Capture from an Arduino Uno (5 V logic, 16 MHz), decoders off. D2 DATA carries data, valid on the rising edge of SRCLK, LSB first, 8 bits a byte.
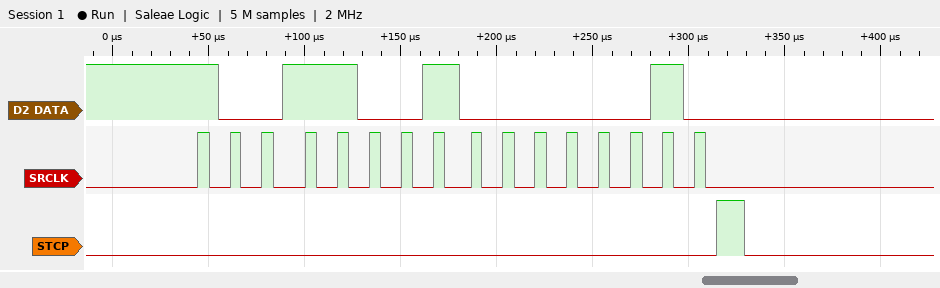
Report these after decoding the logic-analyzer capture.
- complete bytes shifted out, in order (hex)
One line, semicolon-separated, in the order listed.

0x99 0x40
